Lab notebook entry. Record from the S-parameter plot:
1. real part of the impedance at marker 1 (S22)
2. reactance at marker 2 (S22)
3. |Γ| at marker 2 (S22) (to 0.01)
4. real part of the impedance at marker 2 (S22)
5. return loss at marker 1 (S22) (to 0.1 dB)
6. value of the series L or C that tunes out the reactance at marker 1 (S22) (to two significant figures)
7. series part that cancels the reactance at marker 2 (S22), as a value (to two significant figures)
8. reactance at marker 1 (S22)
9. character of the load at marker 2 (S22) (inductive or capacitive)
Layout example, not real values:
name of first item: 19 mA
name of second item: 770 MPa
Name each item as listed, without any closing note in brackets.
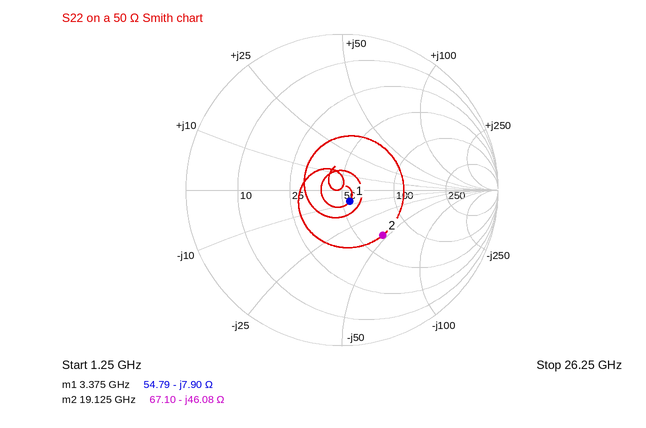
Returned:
real part of the impedance at marker 1: 54.79 Ω
reactance at marker 2: -46.08 Ω
|Γ| at marker 2 (S22): 0.39
real part of the impedance at marker 2: 67.10 Ω
return loss at marker 1 (S22): 21.1 dB
value of the series L or C that tunes out the reactance at marker 1 (S22): 370 pH
series part that cancels the reactance at marker 2 (S22), as a value: 380 pH
reactance at marker 1: -7.90 Ω
character of the load at marker 2 (S22): capacitive
